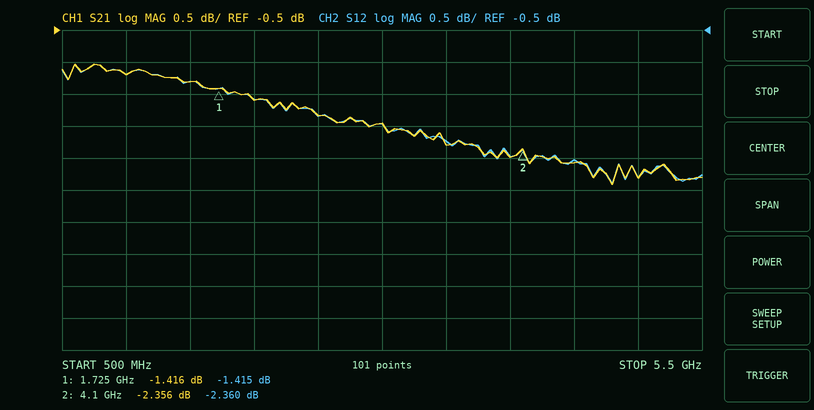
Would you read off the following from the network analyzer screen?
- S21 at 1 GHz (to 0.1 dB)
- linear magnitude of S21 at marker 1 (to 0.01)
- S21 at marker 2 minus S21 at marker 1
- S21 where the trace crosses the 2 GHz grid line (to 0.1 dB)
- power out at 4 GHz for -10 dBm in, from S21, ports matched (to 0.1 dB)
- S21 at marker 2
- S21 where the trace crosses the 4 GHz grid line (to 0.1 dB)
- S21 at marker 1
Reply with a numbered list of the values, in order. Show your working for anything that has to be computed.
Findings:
1. -1.2 dB
2. 10^(-1.416/20) ≈ 0.85
3. -2.356 − (-1.416) = -0.940 dB
4. -1.6 dB
5. -10 dBm + (-2.5 dB) = -12.5 dBm
6. -2.356 dB
7. -2.5 dB
8. -1.416 dB
